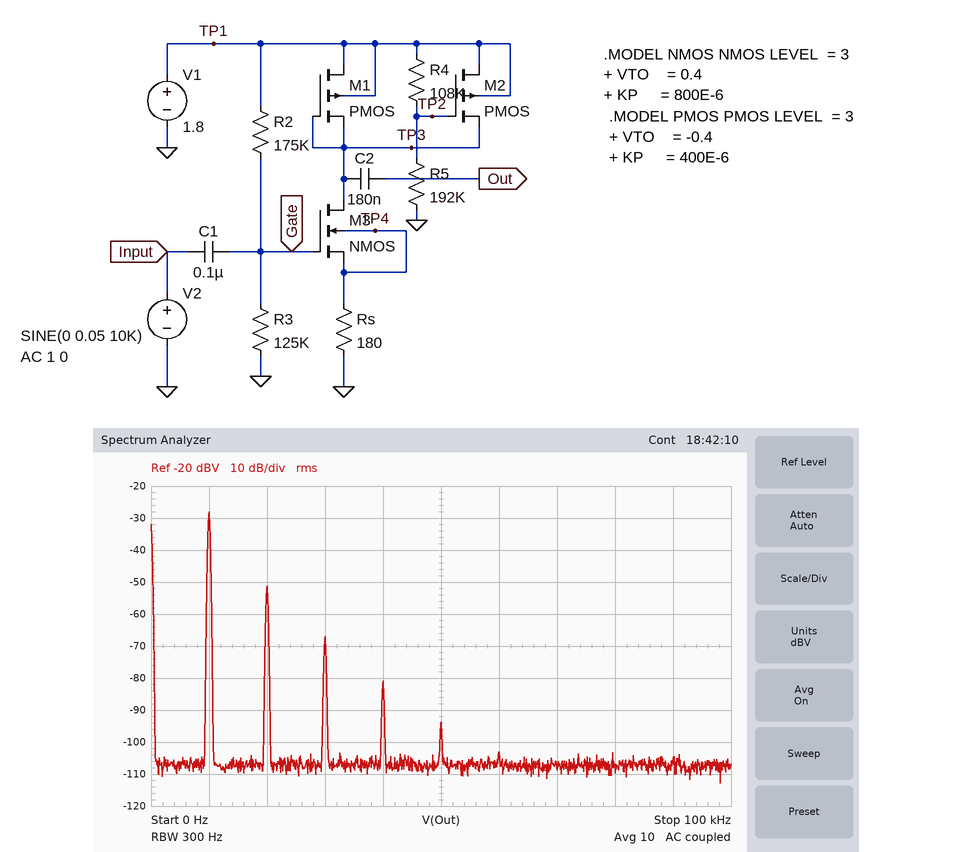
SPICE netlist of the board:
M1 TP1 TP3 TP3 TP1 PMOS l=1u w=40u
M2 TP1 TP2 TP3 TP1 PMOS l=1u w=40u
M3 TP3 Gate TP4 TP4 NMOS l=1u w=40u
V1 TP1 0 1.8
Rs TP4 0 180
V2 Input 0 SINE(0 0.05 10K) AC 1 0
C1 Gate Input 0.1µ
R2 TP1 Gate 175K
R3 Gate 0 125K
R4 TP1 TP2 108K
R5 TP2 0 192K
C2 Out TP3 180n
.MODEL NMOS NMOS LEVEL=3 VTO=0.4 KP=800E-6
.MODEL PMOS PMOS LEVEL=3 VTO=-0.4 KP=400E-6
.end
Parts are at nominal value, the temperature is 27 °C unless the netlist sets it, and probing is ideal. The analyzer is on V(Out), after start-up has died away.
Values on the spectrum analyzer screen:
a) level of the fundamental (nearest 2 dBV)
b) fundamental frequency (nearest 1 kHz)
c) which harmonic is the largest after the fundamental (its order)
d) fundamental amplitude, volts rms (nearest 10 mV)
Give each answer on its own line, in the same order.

-28 dBV
10 kHz
2
40 mV
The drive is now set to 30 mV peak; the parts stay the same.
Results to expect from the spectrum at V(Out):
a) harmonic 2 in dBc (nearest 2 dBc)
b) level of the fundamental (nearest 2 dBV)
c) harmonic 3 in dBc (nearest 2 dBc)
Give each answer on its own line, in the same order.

-28 dBc
-32 dBV
-48 dBc
